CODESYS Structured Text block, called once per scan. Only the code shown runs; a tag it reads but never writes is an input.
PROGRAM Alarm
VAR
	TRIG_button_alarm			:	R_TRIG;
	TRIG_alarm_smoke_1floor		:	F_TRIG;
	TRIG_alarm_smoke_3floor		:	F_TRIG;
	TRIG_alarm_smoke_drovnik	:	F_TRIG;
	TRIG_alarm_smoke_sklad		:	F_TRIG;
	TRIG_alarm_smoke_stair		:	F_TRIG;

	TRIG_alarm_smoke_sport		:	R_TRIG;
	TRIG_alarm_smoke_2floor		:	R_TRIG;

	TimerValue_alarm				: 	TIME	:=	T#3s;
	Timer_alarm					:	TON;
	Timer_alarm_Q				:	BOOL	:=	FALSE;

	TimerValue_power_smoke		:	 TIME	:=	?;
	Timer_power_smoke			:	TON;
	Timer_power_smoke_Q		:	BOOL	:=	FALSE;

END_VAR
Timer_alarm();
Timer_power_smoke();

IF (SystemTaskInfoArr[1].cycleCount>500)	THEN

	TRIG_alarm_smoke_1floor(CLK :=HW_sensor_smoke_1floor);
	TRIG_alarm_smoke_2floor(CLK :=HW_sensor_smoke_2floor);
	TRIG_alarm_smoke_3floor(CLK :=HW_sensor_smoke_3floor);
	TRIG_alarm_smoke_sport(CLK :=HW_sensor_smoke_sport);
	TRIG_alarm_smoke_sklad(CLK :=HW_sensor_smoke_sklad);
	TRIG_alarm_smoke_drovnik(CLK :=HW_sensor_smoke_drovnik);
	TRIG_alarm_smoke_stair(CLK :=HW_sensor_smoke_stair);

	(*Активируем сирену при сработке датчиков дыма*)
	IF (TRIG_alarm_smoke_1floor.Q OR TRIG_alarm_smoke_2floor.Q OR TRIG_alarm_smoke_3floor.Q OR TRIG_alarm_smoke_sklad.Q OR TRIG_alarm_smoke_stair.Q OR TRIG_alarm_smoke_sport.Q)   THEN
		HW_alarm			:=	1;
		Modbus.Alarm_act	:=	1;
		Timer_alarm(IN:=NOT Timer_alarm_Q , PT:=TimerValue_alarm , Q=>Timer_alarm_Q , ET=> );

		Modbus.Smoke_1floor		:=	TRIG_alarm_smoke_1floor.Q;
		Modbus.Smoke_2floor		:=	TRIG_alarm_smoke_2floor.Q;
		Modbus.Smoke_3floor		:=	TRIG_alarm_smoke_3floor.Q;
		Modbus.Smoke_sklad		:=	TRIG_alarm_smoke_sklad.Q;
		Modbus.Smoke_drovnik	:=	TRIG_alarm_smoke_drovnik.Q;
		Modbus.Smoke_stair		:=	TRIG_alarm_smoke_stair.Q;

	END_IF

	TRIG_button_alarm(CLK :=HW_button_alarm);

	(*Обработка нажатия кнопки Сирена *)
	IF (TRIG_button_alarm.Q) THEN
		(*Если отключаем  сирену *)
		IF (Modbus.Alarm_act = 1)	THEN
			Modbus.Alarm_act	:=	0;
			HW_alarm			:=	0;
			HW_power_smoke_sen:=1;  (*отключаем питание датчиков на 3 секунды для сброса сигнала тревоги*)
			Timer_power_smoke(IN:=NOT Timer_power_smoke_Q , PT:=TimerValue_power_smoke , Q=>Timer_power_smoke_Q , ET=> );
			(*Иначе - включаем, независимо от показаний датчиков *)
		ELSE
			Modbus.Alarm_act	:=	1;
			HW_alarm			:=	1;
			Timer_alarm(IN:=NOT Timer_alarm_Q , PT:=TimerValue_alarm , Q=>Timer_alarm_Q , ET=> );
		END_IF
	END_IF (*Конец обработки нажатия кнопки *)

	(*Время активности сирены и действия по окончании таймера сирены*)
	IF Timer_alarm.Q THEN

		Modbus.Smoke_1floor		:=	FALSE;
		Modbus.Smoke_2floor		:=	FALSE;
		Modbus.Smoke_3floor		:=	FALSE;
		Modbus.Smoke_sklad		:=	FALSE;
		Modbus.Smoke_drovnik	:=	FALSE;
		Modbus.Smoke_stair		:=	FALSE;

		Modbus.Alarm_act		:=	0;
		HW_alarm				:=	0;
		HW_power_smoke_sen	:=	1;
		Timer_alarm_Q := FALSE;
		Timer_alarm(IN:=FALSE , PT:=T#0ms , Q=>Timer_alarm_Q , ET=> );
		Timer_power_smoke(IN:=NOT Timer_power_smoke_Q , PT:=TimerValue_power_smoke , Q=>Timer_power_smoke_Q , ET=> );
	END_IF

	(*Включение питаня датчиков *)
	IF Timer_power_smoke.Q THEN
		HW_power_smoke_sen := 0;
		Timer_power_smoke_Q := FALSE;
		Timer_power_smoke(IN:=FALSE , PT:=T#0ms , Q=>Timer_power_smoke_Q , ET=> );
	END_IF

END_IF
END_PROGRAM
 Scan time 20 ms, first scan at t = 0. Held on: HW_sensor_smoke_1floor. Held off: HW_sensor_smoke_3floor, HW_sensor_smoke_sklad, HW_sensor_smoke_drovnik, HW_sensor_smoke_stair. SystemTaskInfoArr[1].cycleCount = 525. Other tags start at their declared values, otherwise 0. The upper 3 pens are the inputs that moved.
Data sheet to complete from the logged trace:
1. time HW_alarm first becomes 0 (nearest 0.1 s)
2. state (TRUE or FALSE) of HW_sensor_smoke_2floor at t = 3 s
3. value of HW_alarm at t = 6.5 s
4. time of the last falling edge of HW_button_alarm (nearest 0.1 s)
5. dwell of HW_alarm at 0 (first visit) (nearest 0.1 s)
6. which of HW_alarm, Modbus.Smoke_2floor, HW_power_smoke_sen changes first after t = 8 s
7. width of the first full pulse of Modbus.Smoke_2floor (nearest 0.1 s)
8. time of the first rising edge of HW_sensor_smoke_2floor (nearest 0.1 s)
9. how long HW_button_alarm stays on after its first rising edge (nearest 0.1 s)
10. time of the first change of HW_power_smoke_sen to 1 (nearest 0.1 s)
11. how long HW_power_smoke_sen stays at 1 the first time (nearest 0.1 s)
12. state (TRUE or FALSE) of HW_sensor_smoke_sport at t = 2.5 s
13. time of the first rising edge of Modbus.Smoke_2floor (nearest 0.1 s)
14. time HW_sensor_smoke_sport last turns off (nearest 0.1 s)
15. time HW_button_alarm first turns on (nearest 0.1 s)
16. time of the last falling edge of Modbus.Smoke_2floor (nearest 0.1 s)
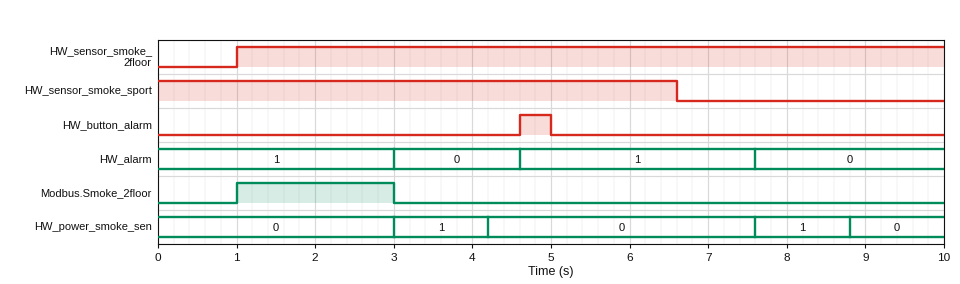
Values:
3.0 s
TRUE
1
5.0 s
1.6 s
HW_power_smoke_sen
2.0 s
1.0 s
0.4 s
3.0 s
1.2 s
TRUE
1.0 s
6.6 s
4.6 s
3.0 s
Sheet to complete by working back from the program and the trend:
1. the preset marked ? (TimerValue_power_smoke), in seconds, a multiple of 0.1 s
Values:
1.2 s
